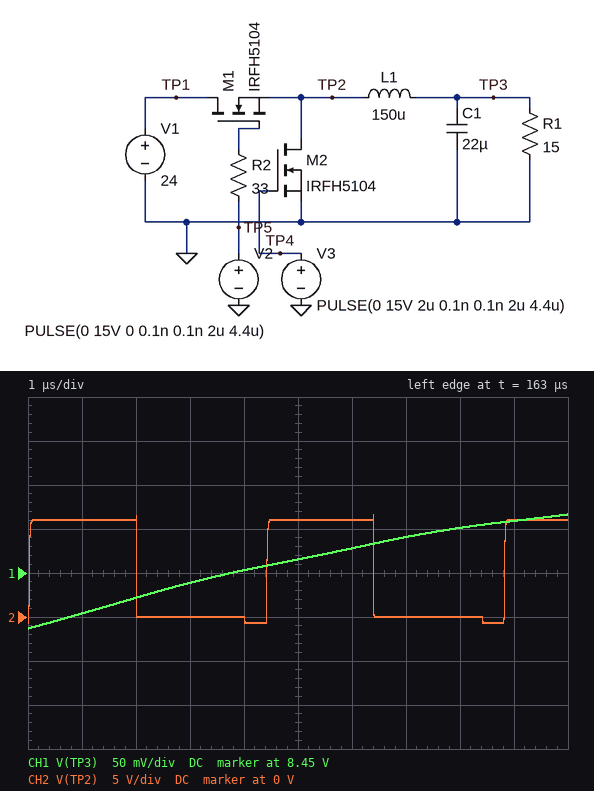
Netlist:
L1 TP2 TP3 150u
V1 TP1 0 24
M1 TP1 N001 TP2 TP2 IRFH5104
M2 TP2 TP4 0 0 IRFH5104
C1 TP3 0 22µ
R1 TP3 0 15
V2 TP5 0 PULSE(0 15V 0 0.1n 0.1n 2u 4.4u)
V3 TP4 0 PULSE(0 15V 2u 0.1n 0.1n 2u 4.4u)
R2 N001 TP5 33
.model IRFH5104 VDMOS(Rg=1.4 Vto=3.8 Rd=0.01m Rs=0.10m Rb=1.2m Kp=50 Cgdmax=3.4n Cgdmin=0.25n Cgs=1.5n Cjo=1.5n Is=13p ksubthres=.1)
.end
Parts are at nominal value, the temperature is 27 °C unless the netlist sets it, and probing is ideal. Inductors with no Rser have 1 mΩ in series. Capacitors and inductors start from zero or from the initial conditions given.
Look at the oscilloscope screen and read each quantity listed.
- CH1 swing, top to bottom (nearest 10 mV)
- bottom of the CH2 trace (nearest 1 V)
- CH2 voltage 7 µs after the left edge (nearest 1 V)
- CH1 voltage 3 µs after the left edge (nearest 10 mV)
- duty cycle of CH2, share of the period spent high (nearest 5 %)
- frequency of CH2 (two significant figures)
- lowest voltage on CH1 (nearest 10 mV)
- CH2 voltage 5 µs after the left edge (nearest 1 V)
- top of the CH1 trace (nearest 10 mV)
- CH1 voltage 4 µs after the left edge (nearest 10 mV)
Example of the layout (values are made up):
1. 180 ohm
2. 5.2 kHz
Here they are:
1. 130 mV
2. -1 V
3. 0 V
4. 8.44 V
5. 45 %
6. 230 kHz
7. 8.39 V
8. 11 V
9. 8.52 V
10. 8.45 V
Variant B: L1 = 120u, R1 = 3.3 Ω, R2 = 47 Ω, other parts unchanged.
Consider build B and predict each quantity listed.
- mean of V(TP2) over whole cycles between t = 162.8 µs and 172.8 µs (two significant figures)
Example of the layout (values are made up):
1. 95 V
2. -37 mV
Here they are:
1. 4.8 V
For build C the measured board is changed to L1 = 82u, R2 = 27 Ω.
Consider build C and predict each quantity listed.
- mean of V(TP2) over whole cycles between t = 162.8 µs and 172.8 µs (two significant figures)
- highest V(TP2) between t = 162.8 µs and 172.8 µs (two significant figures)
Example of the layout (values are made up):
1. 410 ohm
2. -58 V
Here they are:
1. 8.2 V
2. 25 V
